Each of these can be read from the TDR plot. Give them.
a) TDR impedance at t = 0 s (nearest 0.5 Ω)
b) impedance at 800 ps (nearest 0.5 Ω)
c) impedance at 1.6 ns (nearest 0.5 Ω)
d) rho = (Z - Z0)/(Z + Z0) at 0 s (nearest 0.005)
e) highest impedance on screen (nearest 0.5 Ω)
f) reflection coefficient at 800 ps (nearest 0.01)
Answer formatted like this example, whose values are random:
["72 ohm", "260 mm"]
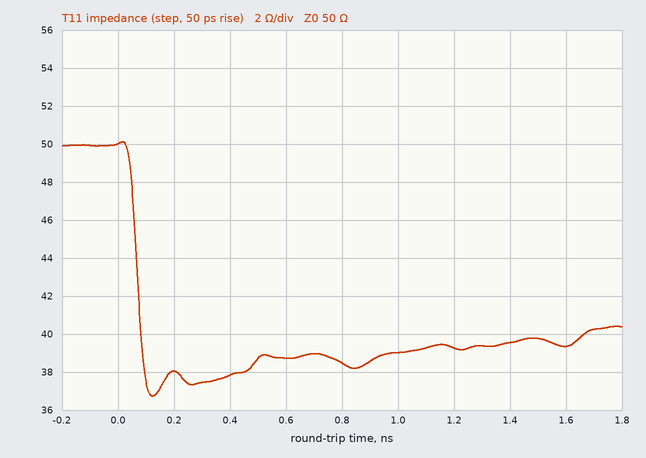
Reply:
["50.0 Ω", "38.5 Ω", "39.5 Ω", "0.000", "50.0 Ω", "-0.13"]
